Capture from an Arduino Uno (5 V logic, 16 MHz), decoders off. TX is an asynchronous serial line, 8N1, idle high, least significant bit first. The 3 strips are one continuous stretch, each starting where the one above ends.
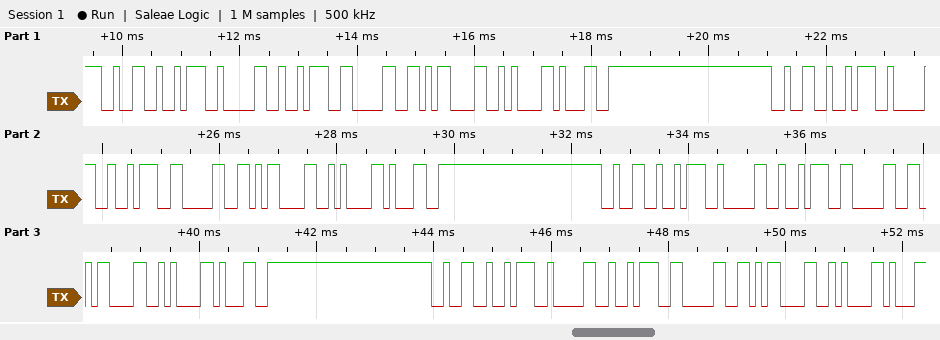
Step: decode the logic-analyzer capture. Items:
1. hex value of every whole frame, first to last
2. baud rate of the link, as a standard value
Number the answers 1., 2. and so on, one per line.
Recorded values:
1. 32 3A 30 3A 30 0D 0A 31 32 3A 30 3A 30 0D 0A 31 32 3A 30 3A 30 0D 0A 31 32 3A 30 3A 30 0D 0A
2. 9600 baud
